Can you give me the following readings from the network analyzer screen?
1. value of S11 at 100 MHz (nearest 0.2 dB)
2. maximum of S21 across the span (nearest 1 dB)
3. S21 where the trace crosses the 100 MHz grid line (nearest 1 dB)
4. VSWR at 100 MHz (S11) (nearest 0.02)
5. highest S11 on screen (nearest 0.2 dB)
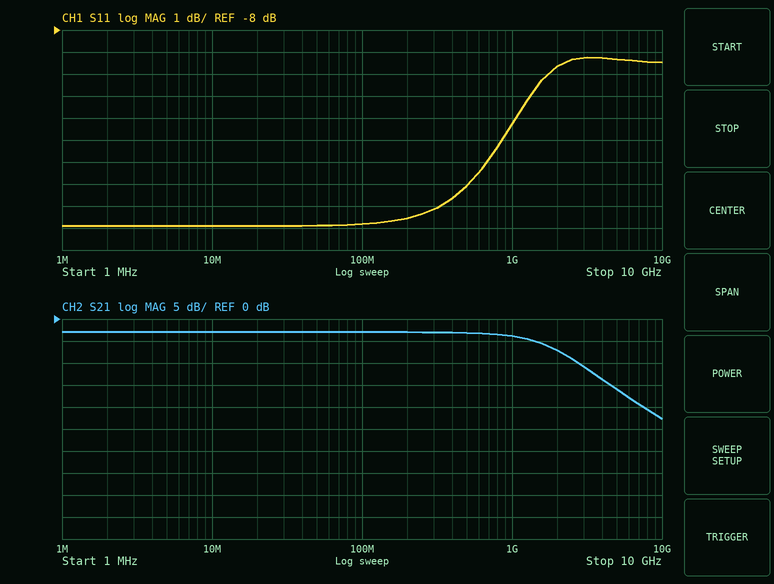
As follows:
-16.8 dB
-3 dB
-3 dB
1.34
-9.2 dB
